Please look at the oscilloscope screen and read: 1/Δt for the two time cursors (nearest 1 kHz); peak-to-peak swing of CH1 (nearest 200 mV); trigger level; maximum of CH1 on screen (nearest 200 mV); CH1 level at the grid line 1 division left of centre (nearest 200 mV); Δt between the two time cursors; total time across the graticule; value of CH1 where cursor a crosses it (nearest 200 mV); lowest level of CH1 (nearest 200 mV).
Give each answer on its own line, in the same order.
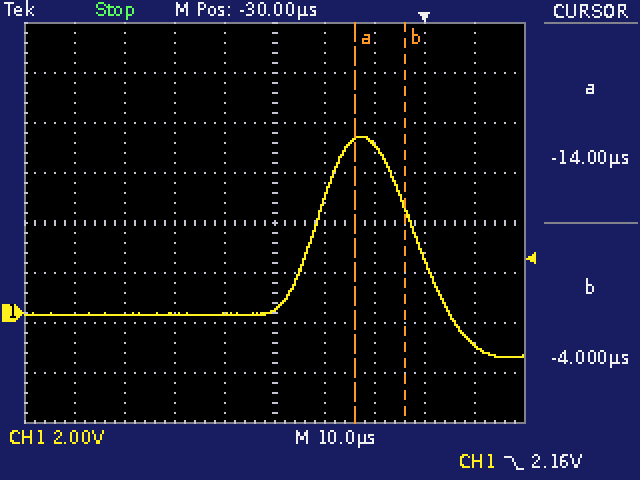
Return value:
100 kHz
8.8 V
2.16 V
7.0 V
0.0 V
10 µs
100 µs
6.8 V
-1.8 V
